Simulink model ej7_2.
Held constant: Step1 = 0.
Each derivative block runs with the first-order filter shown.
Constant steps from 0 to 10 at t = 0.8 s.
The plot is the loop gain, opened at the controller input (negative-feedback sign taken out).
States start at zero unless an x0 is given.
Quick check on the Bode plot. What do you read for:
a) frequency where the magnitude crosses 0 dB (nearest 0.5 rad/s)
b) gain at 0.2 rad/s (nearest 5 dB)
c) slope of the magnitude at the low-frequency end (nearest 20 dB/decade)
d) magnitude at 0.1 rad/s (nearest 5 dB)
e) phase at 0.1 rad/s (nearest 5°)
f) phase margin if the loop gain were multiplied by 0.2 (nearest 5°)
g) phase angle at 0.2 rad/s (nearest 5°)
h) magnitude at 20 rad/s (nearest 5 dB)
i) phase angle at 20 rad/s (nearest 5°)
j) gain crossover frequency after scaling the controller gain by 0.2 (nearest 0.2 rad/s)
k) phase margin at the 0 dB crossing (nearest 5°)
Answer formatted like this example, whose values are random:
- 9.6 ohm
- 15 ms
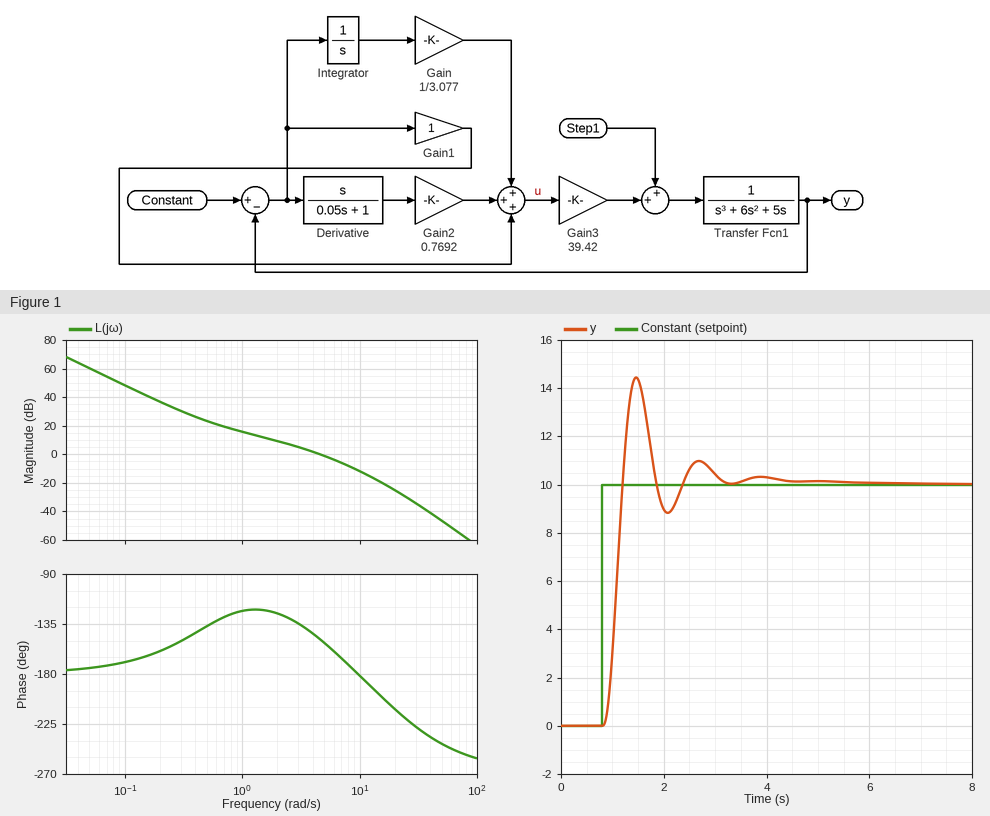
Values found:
- 4.5 rad/s
- 35 dB
- -40 dB/decade
- 50 dB
- -170°
- 60°
- -160°
- -25 dB
- -210°
- 1.2 rad/s
- 30°
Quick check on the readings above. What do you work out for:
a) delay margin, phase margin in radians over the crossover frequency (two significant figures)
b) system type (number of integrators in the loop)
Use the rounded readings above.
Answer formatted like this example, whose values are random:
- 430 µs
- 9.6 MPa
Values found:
- 0.12 s
- 2
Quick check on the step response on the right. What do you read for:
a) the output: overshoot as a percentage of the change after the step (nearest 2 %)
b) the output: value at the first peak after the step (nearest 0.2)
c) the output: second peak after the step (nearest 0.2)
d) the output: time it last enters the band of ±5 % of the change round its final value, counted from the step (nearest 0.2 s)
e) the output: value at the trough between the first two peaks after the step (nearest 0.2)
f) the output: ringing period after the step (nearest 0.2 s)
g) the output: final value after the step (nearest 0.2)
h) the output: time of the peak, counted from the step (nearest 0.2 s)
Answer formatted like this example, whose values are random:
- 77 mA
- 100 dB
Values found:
- 44 %
- 14.4
- 11.0
- 2.2 s
- 8.8
- 1.2 s
- 10.0
- 0.6 s
